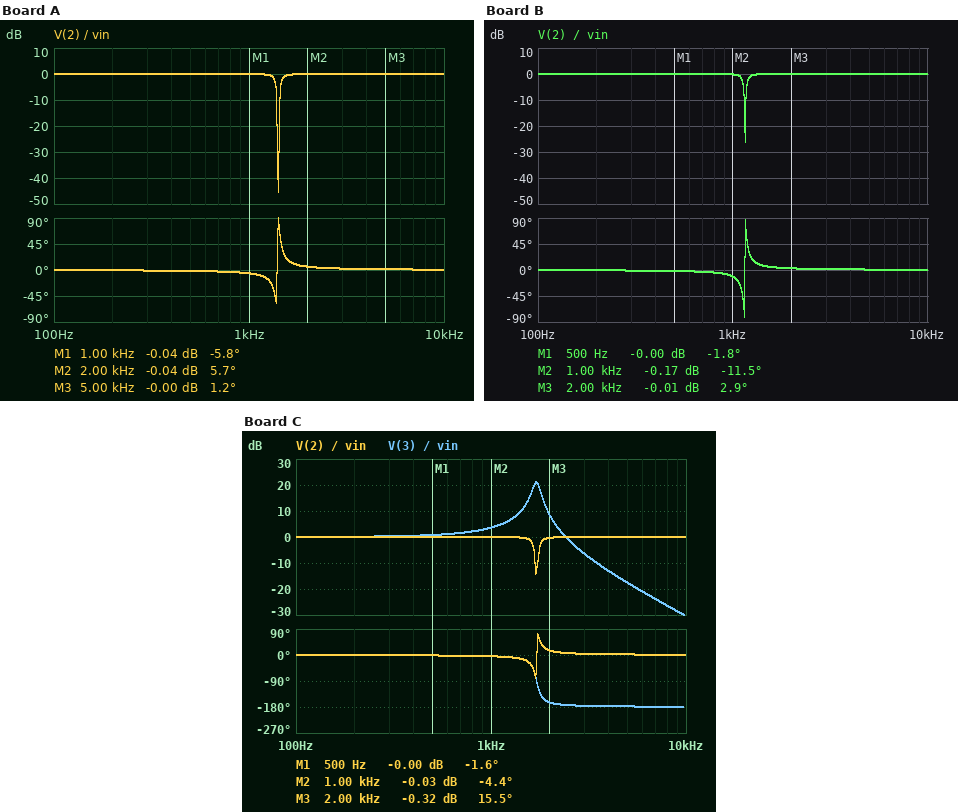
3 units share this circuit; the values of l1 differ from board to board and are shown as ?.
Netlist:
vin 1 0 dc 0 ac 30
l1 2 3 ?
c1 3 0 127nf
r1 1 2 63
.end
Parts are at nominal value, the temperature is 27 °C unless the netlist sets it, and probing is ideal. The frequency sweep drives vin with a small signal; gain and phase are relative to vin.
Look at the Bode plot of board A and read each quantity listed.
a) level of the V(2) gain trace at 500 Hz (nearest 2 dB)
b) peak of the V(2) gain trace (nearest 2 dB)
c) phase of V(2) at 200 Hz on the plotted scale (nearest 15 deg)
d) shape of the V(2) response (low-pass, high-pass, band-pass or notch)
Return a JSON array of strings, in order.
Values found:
["0 dB", "0 dB", "0 deg", "notch"]
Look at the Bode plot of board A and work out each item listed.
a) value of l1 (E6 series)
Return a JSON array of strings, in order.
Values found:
["100 mH"]
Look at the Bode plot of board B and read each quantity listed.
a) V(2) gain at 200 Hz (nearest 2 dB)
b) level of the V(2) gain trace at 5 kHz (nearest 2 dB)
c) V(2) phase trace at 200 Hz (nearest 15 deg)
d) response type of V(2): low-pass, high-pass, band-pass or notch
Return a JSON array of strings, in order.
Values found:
["0 dB", "0 dB", "0 deg", "notch"]
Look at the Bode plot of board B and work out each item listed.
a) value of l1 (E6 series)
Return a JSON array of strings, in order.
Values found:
["150 mH"]
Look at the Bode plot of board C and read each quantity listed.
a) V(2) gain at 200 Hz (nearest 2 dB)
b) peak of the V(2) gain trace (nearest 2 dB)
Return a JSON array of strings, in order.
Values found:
["0 dB", "0 dB"]
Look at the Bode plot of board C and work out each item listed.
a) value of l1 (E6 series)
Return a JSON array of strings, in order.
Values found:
["68 mH"]
